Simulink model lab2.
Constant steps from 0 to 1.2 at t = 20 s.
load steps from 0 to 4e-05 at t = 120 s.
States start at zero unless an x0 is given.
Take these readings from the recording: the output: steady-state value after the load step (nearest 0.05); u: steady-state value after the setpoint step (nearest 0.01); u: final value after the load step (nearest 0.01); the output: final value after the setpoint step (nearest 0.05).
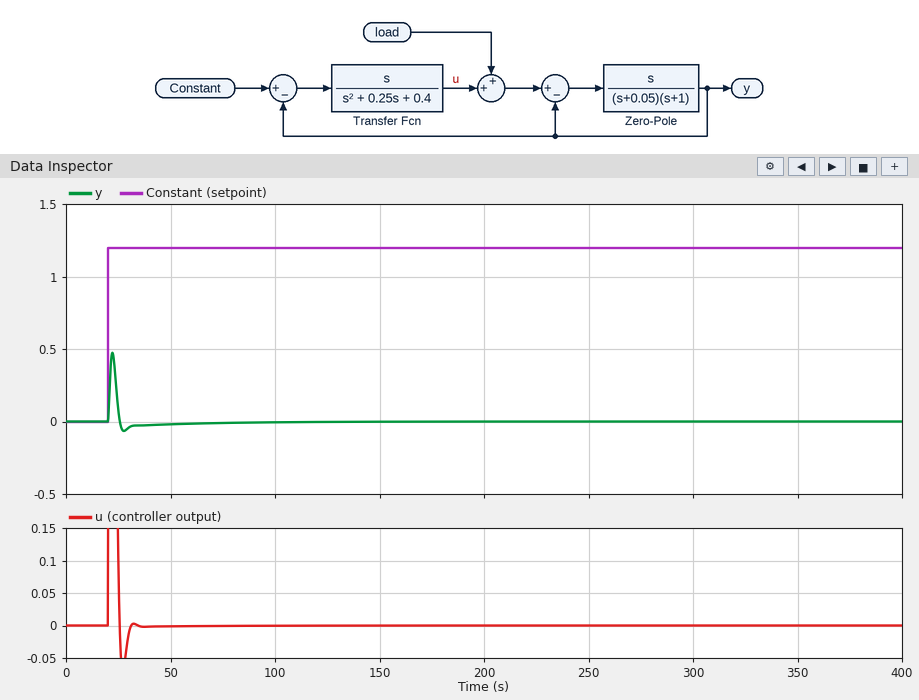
0.00
0.00
0.00
0.00
